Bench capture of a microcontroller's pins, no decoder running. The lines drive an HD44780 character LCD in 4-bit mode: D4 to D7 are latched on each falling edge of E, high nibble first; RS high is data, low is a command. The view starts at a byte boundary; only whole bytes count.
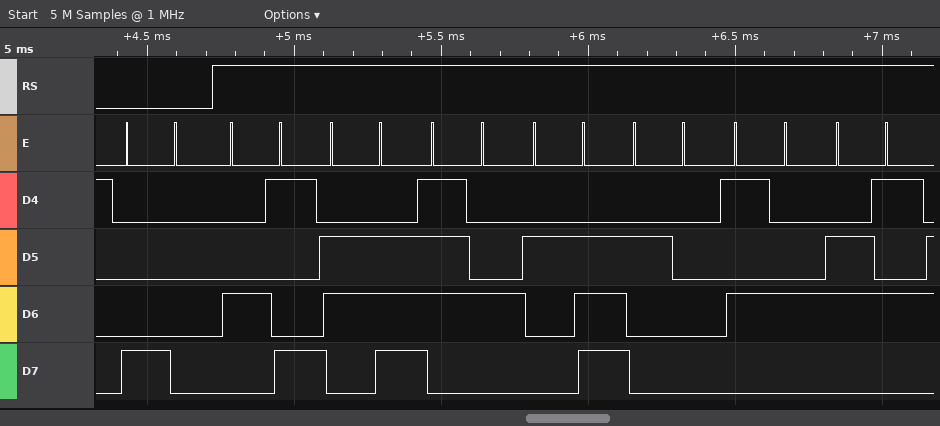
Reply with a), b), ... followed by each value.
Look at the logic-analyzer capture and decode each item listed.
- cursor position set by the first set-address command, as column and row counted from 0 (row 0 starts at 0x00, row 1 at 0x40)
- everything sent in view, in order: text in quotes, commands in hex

a) column 0, row 0
b) 0x80 "Int. Te"
